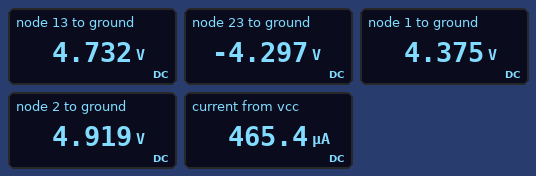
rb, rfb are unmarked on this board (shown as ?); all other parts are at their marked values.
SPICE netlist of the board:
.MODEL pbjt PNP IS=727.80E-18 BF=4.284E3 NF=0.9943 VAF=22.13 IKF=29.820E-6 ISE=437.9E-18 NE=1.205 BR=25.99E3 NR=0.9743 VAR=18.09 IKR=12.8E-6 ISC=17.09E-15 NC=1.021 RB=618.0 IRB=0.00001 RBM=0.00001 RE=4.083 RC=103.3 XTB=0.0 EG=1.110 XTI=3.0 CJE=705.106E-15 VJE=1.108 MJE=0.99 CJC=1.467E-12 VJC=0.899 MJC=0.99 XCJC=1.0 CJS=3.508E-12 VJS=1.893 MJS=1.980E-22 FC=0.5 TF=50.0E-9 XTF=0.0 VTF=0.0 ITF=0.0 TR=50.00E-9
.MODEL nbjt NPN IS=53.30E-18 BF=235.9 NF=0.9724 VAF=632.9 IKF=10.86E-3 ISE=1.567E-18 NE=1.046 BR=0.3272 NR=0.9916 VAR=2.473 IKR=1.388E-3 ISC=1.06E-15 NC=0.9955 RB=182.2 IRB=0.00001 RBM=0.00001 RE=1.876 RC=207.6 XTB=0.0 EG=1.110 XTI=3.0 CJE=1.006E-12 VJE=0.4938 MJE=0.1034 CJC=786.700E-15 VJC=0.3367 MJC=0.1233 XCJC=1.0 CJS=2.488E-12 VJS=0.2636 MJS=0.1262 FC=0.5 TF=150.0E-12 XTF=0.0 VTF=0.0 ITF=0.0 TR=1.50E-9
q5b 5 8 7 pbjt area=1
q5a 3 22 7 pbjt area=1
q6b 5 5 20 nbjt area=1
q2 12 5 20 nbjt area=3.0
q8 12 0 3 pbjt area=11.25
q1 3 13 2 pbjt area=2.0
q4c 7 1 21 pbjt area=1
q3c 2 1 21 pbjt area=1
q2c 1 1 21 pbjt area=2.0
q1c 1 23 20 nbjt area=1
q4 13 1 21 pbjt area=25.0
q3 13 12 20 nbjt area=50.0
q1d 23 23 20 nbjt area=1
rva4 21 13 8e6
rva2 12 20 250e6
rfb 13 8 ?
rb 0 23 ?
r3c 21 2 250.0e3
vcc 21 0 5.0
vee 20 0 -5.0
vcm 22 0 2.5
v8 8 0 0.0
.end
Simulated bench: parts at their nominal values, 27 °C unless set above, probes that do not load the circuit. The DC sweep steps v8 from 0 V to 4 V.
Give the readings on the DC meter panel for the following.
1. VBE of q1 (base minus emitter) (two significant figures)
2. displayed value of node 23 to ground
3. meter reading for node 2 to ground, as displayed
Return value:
-190 mV
-4.297 V
4.919 V
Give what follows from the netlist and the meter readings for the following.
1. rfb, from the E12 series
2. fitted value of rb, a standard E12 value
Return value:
12 kΩ
82 kΩ
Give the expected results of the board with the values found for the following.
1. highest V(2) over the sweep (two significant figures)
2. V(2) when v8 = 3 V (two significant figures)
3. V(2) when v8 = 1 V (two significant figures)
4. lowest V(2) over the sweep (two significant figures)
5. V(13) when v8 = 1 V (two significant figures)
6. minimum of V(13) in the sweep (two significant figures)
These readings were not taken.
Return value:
4.9 V
620 mV
4.9 V
620 mV
4.8 V
-28 mV
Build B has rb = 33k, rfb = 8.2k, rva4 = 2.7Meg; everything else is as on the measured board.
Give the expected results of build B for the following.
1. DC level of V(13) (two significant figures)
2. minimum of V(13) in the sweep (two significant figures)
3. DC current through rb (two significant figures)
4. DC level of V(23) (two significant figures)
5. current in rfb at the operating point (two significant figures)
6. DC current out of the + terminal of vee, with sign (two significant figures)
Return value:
4.8 V
-30 mV
130 µA
-4.3 V
590 µA
-290 µA
